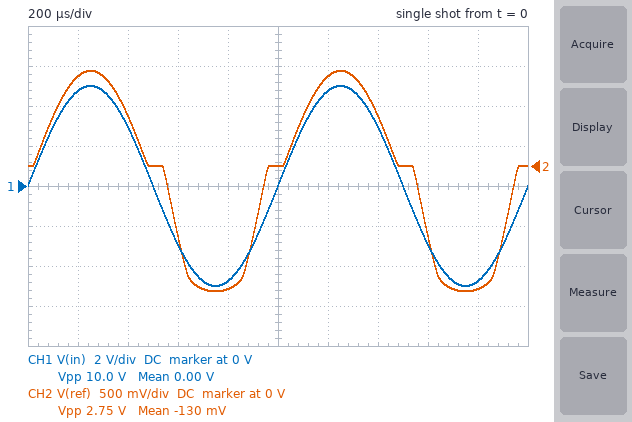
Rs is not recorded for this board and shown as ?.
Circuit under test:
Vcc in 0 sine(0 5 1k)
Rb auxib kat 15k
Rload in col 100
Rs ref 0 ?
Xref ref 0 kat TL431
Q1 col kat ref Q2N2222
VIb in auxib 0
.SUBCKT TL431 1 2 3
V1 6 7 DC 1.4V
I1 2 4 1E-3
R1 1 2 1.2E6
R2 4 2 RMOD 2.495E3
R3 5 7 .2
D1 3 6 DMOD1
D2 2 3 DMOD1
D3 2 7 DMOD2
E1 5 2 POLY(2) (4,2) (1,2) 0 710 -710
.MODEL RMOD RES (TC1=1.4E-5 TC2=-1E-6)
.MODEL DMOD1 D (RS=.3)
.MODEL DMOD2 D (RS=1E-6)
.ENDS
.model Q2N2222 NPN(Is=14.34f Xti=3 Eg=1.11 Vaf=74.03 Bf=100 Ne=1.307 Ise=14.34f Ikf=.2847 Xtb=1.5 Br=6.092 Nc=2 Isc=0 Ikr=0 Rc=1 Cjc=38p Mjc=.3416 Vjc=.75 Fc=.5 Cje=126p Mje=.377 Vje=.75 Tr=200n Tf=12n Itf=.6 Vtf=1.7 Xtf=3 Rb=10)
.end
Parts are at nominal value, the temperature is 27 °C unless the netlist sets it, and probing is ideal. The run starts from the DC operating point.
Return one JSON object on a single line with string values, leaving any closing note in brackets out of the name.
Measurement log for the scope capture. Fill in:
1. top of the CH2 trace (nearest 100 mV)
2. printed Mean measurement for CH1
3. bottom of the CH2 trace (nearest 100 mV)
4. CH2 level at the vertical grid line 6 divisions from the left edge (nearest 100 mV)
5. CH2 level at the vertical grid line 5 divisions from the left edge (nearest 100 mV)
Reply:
{"top of the CH2 trace": "1.2 V", "printed Mean measurement for CH1": "0.00 V", "bottom of the CH2 trace": "-1.6 V", "CH2 level at the vertical grid line 6 divisions from the left edge": "1.1 V", "CH2 level at the vertical grid line 5 divisions from the left edge": "0 V"}
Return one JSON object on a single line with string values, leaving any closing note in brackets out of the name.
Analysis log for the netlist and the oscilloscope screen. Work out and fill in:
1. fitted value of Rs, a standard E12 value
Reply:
{"fitted value of Rs, a standard E12 value": "68 Ω"}
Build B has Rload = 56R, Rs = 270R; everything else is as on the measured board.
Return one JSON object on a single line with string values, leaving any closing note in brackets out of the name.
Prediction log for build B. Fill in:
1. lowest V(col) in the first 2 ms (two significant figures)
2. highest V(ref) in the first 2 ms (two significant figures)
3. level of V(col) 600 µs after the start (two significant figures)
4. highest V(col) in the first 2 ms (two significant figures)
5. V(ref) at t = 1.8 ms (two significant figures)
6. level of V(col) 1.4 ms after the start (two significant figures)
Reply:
{"lowest V(col) in the first 2 ms": "-2.1 V", "highest V(ref) in the first 2 ms": "2.5 V", "level of V(col) 600 µs after the start": "-1.7 V", "highest V(col) in the first 2 ms": "4.5 V", "V(ref) at t = 1.8 ms": "-2.0 V", "level of V(col) 1.4 ms after the start": "2.7 V"}
